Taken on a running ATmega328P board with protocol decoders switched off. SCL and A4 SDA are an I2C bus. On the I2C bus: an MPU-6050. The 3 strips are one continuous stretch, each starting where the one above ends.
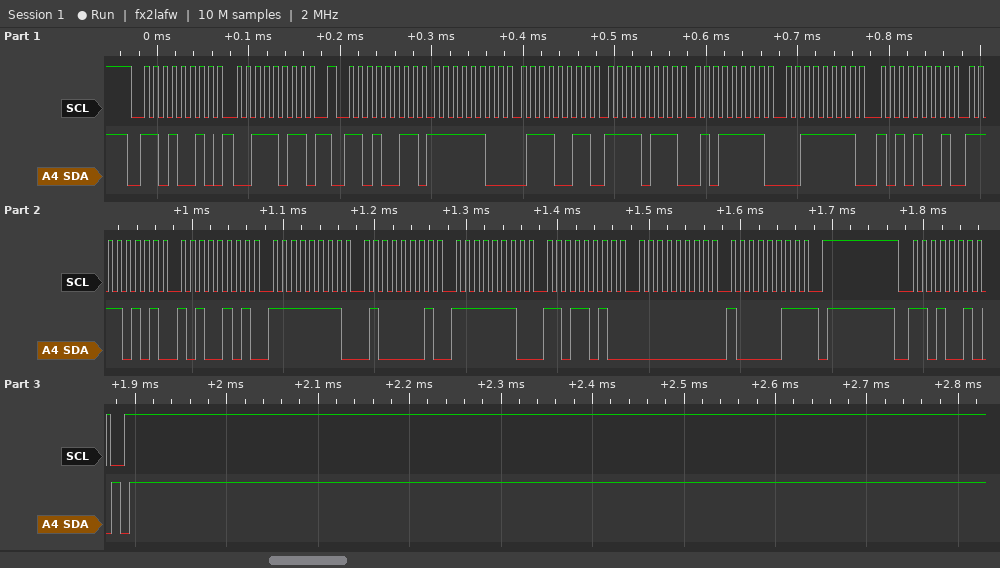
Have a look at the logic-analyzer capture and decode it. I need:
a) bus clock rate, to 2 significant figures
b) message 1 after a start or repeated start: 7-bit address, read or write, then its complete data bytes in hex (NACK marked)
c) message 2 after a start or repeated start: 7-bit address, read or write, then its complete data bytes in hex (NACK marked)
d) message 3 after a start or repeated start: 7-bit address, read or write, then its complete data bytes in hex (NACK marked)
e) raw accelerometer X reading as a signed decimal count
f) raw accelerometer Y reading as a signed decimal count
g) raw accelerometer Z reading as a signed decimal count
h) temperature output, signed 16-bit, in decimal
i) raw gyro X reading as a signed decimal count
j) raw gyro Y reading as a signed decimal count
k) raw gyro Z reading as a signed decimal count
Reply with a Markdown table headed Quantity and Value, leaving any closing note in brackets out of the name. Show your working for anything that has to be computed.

| Quantity | Value |
|---|---|
| bus clock rate, to 2 significant figures | 100 kHz |
| message 1 after a start or repeated start: 7-bit address, read or write, then its complete data bytes in hex | 0x69 write: 3B |
| message 2 after a start or repeated start: 7-bit address, read or write, then its complete data bytes in hex | 0x69 read: FC 73 F7 5F 3F A9 F5 A5 FF 41 FE DA 00 83 NACK |
| message 3 after a start or repeated start: 7-bit address, read or write, then its complete data bytes in hex | 0x69 write |
| raw accelerometer X reading as a signed decimal count | 0xFC73 = -909 |
| raw accelerometer Y reading as a signed decimal count | 0xF75F = -2209 |
| raw accelerometer Z reading as a signed decimal count | 0x3FA9 = 16297 |
| temperature output, signed 16-bit, in decimal | 0xF5A5 = -2651 |
| raw gyro X reading as a signed decimal count | 0xFF41 = -191 |
| raw gyro Y reading as a signed decimal count | 0xFEDA = -294 |
| raw gyro Z reading as a signed decimal count | 0x0083 = 131 |
